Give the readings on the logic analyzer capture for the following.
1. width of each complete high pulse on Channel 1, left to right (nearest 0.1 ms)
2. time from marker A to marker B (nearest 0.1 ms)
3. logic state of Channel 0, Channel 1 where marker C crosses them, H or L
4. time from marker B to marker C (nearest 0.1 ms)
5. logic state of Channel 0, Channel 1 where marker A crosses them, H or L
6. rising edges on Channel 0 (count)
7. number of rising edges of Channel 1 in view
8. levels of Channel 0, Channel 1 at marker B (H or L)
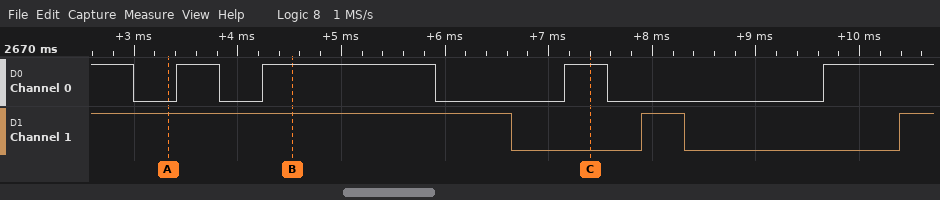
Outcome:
0.4 ms
1.2 ms
Channel 0=H, Channel 1=L
2.9 ms
Channel 0=L, Channel 1=H
4
2
Channel 0=H, Channel 1=H
